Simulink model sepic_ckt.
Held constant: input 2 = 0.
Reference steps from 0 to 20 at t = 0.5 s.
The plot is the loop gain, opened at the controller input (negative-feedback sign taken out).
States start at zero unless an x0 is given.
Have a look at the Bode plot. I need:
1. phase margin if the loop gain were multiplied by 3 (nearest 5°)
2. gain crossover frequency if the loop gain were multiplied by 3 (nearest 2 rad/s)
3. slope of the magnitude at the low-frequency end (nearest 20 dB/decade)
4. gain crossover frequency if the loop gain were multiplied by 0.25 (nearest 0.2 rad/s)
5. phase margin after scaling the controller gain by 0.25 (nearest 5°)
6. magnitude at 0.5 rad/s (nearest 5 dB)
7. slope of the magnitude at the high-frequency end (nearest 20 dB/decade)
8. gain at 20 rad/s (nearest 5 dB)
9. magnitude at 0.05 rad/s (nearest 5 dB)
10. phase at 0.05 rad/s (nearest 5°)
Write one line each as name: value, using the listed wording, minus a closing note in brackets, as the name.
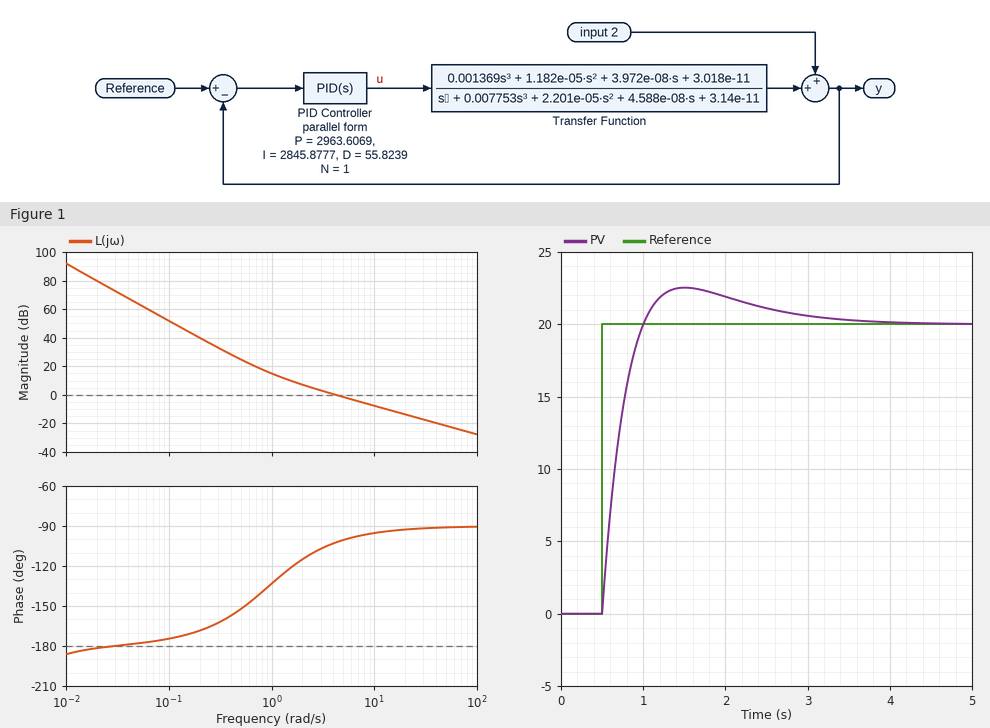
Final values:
phase margin if the loop gain were multiplied by 3: 85°
gain crossover frequency if the loop gain were multiplied by 3: 12 rad/s
slope of the magnitude at the low-frequency end: -40 dB/decade
gain crossover frequency if the loop gain were multiplied by 0.25: 1.2 rad/s
phase margin after scaling the controller gain by 0.25: 55°
magnitude at 0.5 rad/s: 25 dB
slope of the magnitude at the high-frequency end: -20 dB/decade
gain at 20 rad/s: -15 dB
magnitude at 0.05 rad/s: 65 dB
phase at 0.05 rad/s: -180°
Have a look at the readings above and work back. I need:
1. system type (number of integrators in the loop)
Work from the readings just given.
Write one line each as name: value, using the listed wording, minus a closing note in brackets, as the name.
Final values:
system type: 2
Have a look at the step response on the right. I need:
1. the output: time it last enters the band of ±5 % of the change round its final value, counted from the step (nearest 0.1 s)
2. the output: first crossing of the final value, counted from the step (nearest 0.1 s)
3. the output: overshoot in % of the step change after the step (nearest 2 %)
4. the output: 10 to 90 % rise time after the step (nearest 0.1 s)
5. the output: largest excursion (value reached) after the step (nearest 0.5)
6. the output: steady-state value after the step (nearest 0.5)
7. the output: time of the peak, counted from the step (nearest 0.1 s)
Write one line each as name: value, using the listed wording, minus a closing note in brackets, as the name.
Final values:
the output: time it last enters the band of ±5 % of the change round its final value, counted from the step: 2.1 s
the output: first crossing of the final value, counted from the step: 0.5 s
the output: overshoot in % of the step change after the step: 12 %
the output: 10 to 90 % rise time after the step: 0.4 s
the output: largest excursion (value reached) after the step: 22.5
the output: steady-state value after the step: 20.0
the output: time of the peak, counted from the step: 1.0 s
